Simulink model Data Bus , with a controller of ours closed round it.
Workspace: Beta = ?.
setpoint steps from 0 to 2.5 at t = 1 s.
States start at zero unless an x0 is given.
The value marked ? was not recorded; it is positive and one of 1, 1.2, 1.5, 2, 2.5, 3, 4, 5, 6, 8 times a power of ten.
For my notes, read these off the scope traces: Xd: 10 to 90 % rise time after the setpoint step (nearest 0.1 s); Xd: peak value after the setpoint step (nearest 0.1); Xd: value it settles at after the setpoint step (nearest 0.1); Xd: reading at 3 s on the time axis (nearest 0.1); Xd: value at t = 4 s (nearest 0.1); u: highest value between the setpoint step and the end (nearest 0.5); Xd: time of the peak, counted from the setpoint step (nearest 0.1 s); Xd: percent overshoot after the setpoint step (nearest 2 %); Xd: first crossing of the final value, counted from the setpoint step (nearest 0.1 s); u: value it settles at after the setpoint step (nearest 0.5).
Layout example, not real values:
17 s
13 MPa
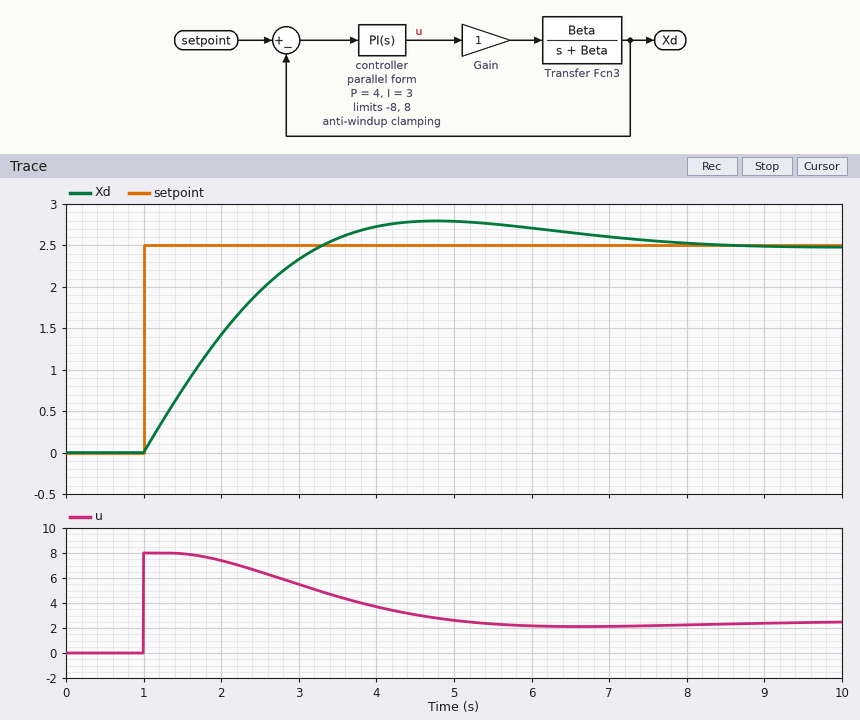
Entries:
1.7 s
2.8
2.5
2.3
2.7
8.0
3.8 s
12 %
2.3 s
2.5
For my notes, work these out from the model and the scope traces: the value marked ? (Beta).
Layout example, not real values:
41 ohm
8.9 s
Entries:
0.2
